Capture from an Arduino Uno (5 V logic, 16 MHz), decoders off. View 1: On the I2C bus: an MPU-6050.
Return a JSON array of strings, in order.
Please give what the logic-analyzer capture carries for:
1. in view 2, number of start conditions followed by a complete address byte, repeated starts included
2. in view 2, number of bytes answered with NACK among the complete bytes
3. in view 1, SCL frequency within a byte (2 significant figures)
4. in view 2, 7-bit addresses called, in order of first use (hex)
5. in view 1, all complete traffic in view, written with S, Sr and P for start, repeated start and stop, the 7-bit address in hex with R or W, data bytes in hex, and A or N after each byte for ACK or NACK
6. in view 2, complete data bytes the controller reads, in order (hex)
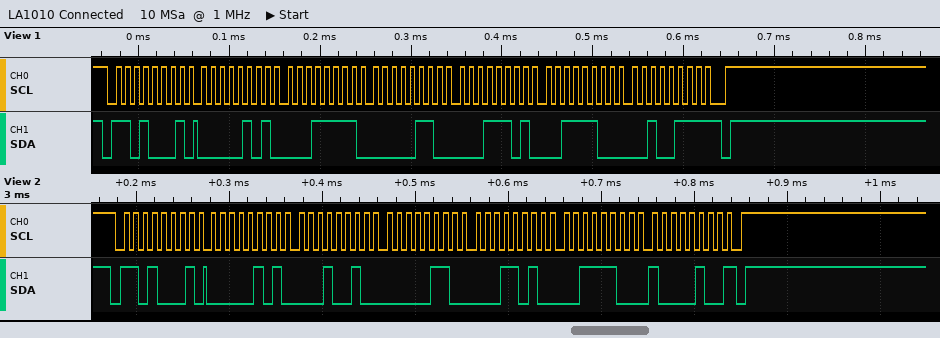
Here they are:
["1", "1", "100 kHz", "0x68", "S 68R A 05 A 1F A 06 A 1D A 3C A 27 N P", "05 12 06 1A 3C 84"]
